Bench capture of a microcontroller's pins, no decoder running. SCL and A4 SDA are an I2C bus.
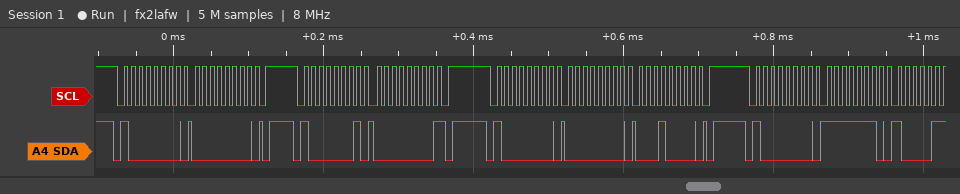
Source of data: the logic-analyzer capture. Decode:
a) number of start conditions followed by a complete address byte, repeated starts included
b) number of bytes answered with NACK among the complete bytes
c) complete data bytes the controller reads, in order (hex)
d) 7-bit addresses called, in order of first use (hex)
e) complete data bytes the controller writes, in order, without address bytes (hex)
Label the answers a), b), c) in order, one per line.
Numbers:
a) 4
b) 1
c) 00
d) 0x40
e) 00 00 10 FE
